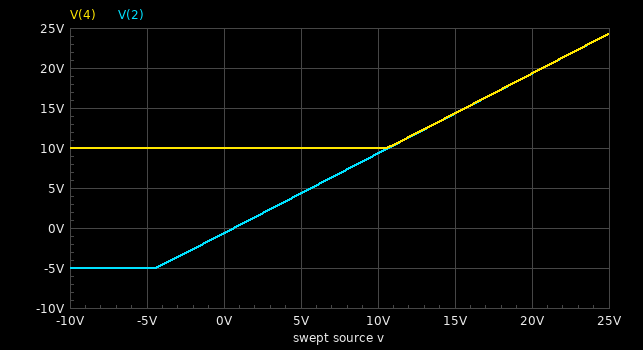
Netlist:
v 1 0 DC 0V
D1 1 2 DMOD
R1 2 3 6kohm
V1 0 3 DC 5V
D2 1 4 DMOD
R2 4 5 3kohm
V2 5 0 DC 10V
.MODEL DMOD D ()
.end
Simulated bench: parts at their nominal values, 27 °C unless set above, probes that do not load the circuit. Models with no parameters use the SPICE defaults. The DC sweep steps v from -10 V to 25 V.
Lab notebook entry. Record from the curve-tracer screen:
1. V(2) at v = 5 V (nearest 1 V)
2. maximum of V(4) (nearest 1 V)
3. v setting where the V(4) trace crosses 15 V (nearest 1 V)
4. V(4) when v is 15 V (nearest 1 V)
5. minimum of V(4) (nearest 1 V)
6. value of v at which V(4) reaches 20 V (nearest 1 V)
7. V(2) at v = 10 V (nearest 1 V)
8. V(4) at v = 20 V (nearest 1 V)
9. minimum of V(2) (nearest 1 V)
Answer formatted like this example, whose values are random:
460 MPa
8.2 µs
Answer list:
4 V
24 V
16 V
14 V
10 V
21 V
9 V
19 V
-5 V
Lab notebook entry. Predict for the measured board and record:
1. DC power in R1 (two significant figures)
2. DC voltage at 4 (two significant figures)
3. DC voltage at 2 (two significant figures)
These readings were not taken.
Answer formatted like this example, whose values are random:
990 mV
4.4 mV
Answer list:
3.2 mW
10 V
-650 mV
